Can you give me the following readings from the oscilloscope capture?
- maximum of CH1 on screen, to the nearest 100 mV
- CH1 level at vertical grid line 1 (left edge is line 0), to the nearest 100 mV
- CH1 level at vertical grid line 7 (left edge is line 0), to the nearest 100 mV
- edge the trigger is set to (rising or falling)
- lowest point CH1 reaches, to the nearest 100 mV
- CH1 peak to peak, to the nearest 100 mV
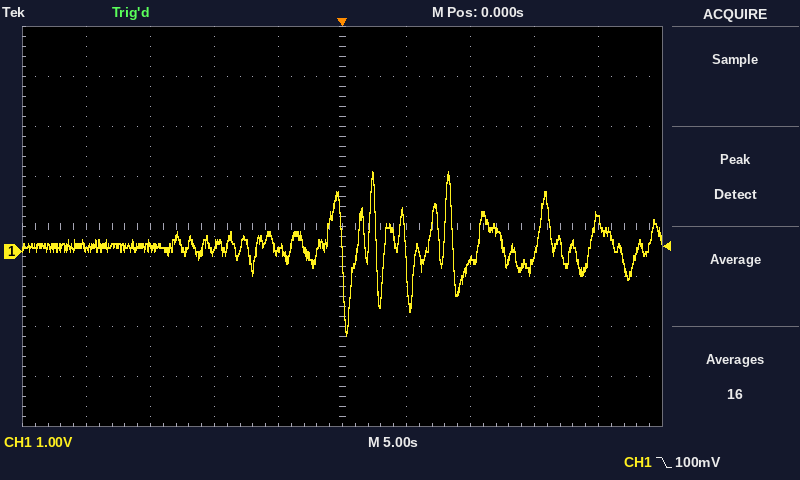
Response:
1.6 V
100 mV
-200 mV
falling
-1.7 V
3.3 V
